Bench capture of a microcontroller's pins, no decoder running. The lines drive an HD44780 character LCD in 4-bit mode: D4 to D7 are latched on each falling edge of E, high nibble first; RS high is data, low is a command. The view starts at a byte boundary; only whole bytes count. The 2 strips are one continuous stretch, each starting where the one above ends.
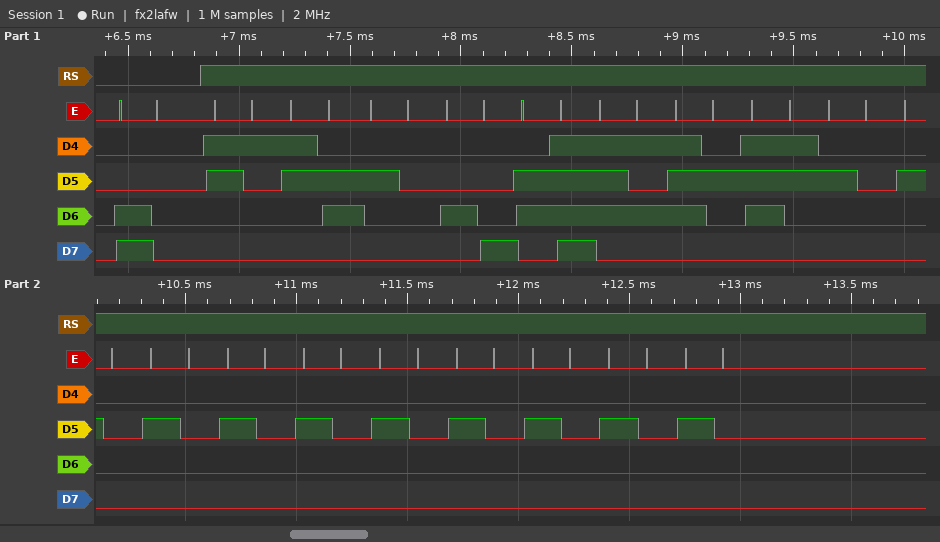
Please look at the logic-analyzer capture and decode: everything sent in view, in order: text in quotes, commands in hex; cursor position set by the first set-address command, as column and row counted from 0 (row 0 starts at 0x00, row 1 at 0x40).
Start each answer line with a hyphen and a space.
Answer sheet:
- 0xC0 "16 Hours          "
- column 0, row 1
